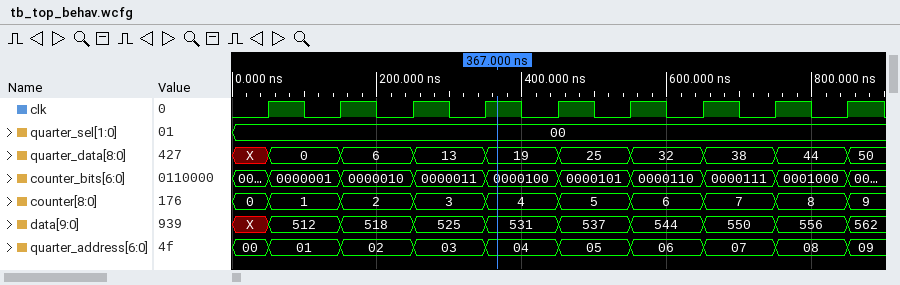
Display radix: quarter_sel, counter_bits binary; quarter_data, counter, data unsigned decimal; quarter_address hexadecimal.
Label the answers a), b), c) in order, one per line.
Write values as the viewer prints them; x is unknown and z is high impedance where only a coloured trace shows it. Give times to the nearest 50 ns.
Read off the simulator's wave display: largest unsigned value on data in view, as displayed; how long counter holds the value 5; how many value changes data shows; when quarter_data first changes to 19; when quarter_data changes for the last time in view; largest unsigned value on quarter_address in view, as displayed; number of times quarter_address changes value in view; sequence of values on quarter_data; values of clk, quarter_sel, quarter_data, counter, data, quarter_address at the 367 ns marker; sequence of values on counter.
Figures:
a) 562
b) 100 ns
c) 9
d) 350 ns
e) 850 ns
f) 09
g) 9
h) X, 0, 6, 13, 19, 25, 32, 38, 44, 50
i) clk=1, quarter_sel=00, quarter_data=19, counter=4, data=531, quarter_address=04
j) 0, 1, 2, 3, 4, 5, 6, 7, 8, 9
